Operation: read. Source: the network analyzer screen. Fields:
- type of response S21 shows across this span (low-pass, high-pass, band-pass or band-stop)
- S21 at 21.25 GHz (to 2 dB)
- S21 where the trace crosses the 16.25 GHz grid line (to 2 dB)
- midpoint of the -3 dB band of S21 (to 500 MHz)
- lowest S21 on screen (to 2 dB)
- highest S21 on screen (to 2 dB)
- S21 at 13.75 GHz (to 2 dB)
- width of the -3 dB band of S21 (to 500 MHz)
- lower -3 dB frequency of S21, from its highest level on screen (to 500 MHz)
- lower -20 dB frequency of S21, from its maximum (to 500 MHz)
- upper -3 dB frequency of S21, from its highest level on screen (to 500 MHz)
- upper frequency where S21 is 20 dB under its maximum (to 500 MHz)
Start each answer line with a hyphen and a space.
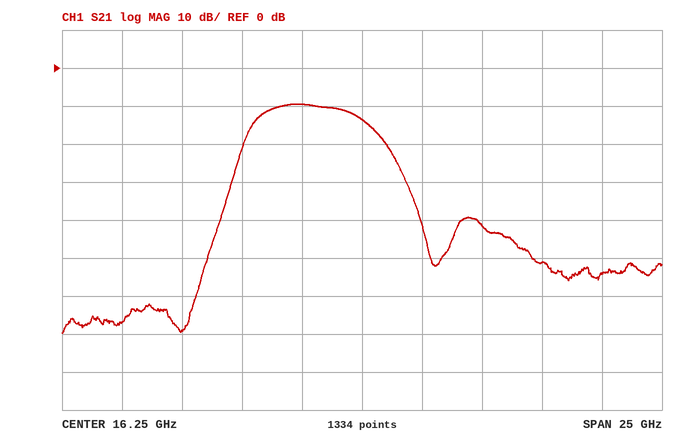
- band-pass
- -42 dB
- -14 dB
- 14.0 GHz
- -70 dB
- -10 dB
- -10 dB
- 4.0 GHz
- 12.0 GHz
- 11.0 GHz
- 16.0 GHz
- 18.0 GHz
